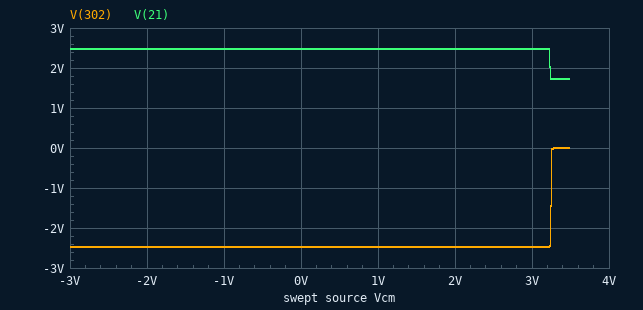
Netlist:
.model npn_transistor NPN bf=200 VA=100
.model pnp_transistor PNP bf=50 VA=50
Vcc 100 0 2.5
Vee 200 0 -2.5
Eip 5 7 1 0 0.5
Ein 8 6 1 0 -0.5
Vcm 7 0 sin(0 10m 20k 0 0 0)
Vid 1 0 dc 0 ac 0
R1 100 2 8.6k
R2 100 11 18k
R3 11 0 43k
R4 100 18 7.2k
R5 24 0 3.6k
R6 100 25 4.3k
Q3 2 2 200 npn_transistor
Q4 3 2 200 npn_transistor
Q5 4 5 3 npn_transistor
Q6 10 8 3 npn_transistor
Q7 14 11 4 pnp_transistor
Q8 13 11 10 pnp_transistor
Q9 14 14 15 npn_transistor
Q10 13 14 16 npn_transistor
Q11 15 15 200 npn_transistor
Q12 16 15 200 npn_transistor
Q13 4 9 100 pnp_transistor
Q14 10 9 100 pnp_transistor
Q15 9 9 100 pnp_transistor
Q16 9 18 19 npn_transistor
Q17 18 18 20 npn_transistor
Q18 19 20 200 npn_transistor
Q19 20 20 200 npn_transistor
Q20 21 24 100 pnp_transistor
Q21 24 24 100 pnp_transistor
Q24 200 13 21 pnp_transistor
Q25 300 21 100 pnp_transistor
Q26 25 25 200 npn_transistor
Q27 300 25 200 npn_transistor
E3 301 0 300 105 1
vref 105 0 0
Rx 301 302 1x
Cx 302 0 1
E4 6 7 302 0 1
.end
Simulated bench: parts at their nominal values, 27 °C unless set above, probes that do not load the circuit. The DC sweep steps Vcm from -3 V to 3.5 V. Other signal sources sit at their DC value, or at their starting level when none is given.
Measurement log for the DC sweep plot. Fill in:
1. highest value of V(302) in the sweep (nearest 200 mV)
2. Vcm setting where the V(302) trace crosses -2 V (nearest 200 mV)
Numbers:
0 V
3.2 V
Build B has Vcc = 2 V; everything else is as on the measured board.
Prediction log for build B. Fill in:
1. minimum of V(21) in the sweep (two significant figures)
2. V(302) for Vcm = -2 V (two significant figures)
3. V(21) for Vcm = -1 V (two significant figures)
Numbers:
1.2 V
-2.5 V
2.0 V
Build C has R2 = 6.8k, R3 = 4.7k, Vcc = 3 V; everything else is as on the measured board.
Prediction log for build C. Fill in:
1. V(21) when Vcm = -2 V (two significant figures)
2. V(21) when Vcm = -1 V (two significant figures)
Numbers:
2.8 V
3.0 V
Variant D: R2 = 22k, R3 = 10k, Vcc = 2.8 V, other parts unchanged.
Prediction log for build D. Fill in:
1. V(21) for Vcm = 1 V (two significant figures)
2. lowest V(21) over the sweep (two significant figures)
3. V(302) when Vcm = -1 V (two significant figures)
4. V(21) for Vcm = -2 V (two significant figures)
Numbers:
2.8 V
2.0 V
-2.5 V
2.6 V
